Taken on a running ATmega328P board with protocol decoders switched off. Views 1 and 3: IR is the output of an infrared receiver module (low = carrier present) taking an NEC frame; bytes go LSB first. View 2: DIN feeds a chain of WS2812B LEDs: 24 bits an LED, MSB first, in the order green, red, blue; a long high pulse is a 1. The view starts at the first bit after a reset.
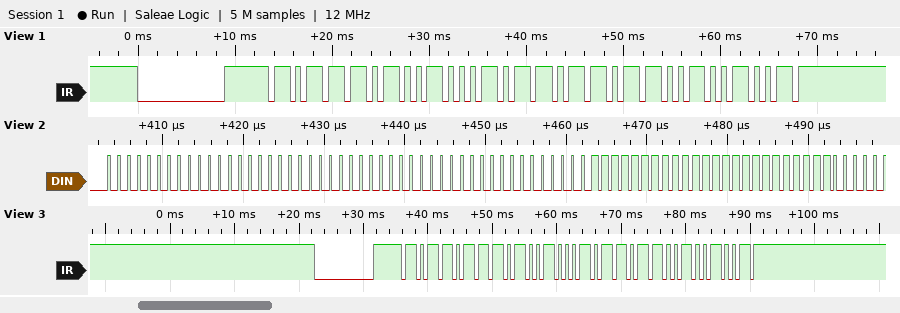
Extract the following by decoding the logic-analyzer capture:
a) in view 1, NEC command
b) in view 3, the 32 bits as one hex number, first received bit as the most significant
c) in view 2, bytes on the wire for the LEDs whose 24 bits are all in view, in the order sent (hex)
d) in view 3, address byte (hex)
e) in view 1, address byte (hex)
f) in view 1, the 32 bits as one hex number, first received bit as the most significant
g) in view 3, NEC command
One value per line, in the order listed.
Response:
0x6D
0xB748B649
00 00 00 00 00 00 FF FF FF
0xED
0x5D
0xBA45B649
0x6D
